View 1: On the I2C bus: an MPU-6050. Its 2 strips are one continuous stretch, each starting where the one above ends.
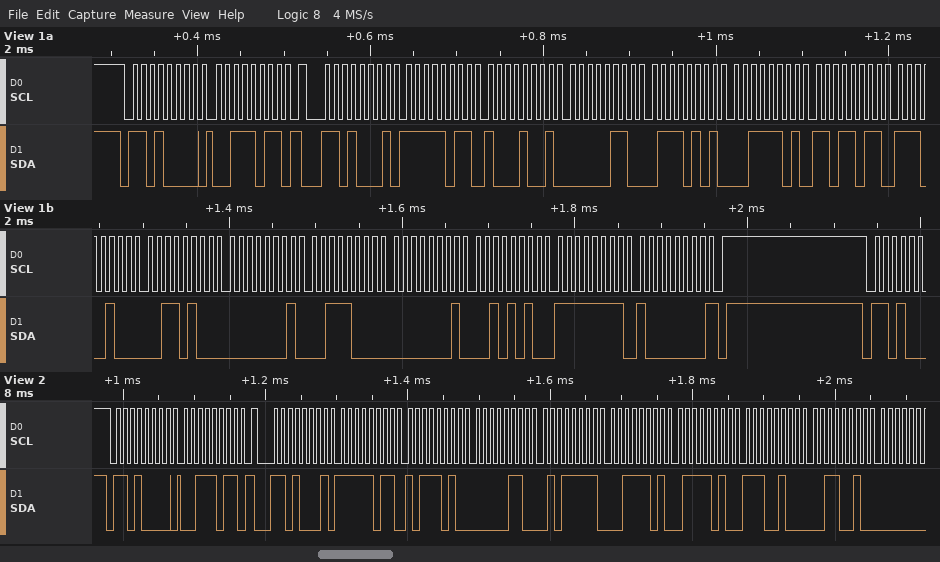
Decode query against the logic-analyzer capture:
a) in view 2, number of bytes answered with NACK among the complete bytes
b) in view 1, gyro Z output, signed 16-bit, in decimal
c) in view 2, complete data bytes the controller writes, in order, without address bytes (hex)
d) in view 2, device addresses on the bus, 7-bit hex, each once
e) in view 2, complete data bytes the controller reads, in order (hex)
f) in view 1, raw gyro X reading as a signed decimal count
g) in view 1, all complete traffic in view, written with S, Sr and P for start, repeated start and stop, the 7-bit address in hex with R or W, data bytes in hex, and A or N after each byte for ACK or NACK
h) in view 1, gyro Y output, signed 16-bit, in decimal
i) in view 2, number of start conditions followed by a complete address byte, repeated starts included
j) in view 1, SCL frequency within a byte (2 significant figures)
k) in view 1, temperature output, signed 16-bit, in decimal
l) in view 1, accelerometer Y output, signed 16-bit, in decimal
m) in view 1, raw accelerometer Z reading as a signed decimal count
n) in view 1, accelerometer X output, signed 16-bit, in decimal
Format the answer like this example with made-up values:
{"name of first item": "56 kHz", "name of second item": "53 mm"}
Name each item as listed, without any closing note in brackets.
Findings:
{"in view 2, number of bytes answered with NACK among the complete bytes": "0", "in view 1, gyro Z output, signed 16-bit, in decimal": "-128", "in view 2, complete data bytes the controller writes, in order, without address bytes": "3B", "in view 2, device addresses on the bus, 7-bit hex, each once": "0x68", "in view 2, complete data bytes the controller reads, in order": "FB BA 06 5F 3D 7A E4 32", "in view 1, raw gyro X reading as a signed decimal count": "312", "in view 1, all complete traffic in view, written with S, Sr and P for start, repeated start and stop, the 7-bit address in hex with R or W, data bytes in hex, and A or N after each byte for ACK or NACK": "S 68W A 3B A Sr 68R A FB A 89 A 06 A 75 A 3D A DB A E4 A 34 A 01 A 38 A 01 A 2A A FF A 80 N P", "in view 1, gyro Y output, signed 16-bit, in decimal": "298", "in view 2, number of start conditions followed by a complete address byte, repeated starts included": "2", "in view 1, SCL frequency within a byte": "100 kHz", "in view 1, temperature output, signed 16-bit, in decimal": "-7116", "in view 1, accelerometer Y output, signed 16-bit, in decimal": "1653", "in view 1, raw accelerometer Z reading as a signed decimal count": "15835", "in view 1, accelerometer X output, signed 16-bit, in decimal": "-1143"}
